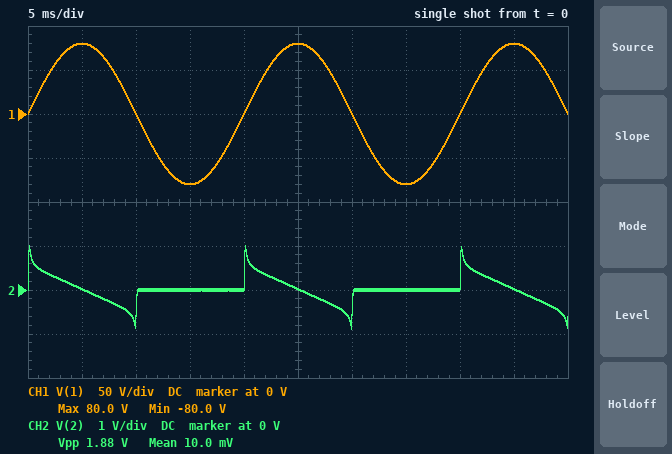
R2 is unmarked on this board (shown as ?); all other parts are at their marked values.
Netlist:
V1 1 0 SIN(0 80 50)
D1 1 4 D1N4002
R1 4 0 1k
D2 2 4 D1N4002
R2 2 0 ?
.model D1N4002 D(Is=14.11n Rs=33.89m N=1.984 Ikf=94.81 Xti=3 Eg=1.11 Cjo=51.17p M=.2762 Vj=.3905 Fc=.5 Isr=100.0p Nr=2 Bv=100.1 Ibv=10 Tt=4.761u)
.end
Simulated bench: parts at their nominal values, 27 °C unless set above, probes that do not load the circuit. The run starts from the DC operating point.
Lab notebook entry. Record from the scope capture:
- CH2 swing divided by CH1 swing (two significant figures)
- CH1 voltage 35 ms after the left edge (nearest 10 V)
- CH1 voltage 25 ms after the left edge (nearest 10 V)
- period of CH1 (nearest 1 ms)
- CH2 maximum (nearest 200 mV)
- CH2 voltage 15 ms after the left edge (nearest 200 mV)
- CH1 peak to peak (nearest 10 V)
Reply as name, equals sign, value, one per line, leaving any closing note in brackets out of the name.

CH2 swing divided by CH1 swing = 0.012
CH1 voltage 35 ms after the left edge = -80 V
CH1 voltage 25 ms after the left edge = 80 V
period of CH1 = 20 ms
CH2 maximum = 1.0 V
CH2 voltage 15 ms after the left edge = 0 V
CH1 peak to peak = 160 V
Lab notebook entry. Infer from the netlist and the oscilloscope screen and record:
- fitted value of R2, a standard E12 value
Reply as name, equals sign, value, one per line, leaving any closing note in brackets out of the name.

fitted value of R2, a standard E12 value = 1.2 MΩ
